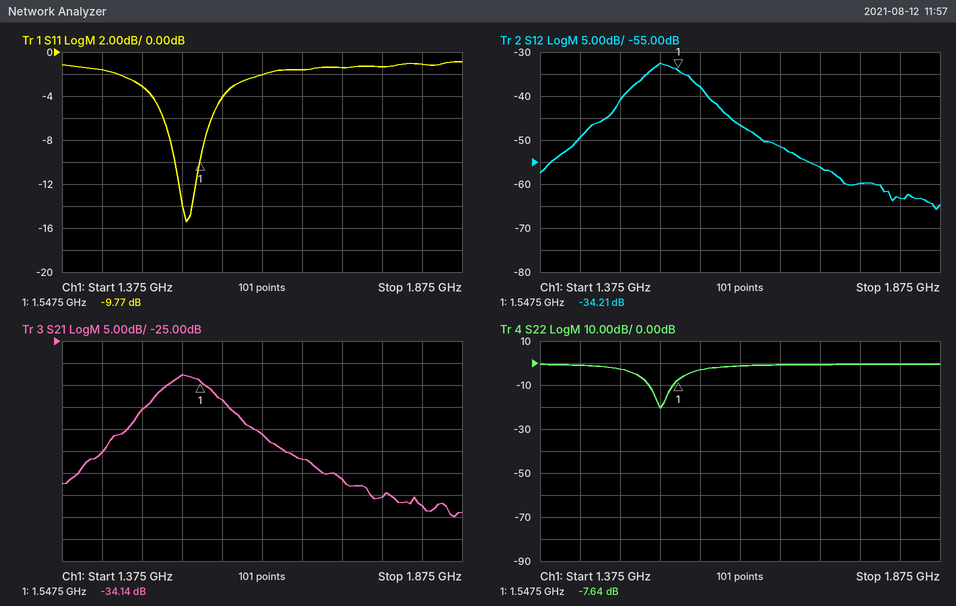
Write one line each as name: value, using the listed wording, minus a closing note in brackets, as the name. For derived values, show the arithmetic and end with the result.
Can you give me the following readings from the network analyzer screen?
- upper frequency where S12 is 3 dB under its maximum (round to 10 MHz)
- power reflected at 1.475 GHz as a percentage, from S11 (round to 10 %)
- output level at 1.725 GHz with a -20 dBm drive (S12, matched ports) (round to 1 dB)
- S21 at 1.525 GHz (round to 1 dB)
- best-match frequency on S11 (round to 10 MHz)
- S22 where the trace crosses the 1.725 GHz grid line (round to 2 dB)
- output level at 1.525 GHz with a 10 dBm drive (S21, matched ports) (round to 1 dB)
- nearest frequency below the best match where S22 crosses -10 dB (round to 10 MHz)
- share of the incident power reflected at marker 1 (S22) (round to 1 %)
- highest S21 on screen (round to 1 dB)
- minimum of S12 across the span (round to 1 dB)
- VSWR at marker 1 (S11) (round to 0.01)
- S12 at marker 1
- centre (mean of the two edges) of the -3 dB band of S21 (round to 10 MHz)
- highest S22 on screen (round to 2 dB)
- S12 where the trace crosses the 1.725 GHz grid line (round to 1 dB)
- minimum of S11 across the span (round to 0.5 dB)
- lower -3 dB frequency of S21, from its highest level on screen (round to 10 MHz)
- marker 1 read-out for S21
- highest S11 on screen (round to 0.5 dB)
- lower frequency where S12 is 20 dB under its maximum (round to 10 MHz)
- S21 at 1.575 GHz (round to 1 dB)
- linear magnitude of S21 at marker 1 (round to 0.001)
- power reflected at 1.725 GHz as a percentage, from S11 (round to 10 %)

upper frequency where S12 is 3 dB under its maximum: 1.56 GHz
power reflected at 1.475 GHz as a percentage, from S11: 10^(-3/10) ≈ 50 %
output level at 1.725 GHz with a -20 dBm drive (S12, matched ports): -20 dBm + (-56 dB) = -76 dBm
S21 at 1.525 GHz: -33 dB
best-match frequency on S11: 1.53 GHz
S22 where the trace crosses the 1.725 GHz grid line: 0 dB
output level at 1.525 GHz with a 10 dBm drive (S21, matched ports): 10 dBm + (-33 dB) = -23 dBm
nearest frequency below the best match where S22 crosses -10 dB: 1.51 GHz
share of the incident power reflected at marker 1 (S22): 10^(-7.64/10) ≈ 17 %
highest S21 on screen: -33 dB
minimum of S12 across the span: -66 dB
VSWR at marker 1 (S11): (1 + 0.3247)/(1 − 0.3247) ≈ 1.96
S12 at marker 1: -34.21 dB
centre (mean of the two edges) of the -3 dB band of S21: 1.53 GHz
highest S22 on screen: 0 dB
S12 where the trace crosses the 1.725 GHz grid line: -56 dB
minimum of S11 across the span: -15.5 dB
lower -3 dB frequency of S21, from its highest level on screen: 1.50 GHz
marker 1 read-out for S21: -34.14 dB
highest S11 on screen: -1.0 dB
lower frequency where S12 is 20 dB under its maximum: 1.41 GHz
S21 at 1.575 GHz: -38 dB
linear magnitude of S21 at marker 1: 10^(-34.14/20) ≈ 0.020
power reflected at 1.725 GHz as a percentage, from S11: 10^(-1.5/10) ≈ 70.8 %, so 70 % to the nearest 10 %
